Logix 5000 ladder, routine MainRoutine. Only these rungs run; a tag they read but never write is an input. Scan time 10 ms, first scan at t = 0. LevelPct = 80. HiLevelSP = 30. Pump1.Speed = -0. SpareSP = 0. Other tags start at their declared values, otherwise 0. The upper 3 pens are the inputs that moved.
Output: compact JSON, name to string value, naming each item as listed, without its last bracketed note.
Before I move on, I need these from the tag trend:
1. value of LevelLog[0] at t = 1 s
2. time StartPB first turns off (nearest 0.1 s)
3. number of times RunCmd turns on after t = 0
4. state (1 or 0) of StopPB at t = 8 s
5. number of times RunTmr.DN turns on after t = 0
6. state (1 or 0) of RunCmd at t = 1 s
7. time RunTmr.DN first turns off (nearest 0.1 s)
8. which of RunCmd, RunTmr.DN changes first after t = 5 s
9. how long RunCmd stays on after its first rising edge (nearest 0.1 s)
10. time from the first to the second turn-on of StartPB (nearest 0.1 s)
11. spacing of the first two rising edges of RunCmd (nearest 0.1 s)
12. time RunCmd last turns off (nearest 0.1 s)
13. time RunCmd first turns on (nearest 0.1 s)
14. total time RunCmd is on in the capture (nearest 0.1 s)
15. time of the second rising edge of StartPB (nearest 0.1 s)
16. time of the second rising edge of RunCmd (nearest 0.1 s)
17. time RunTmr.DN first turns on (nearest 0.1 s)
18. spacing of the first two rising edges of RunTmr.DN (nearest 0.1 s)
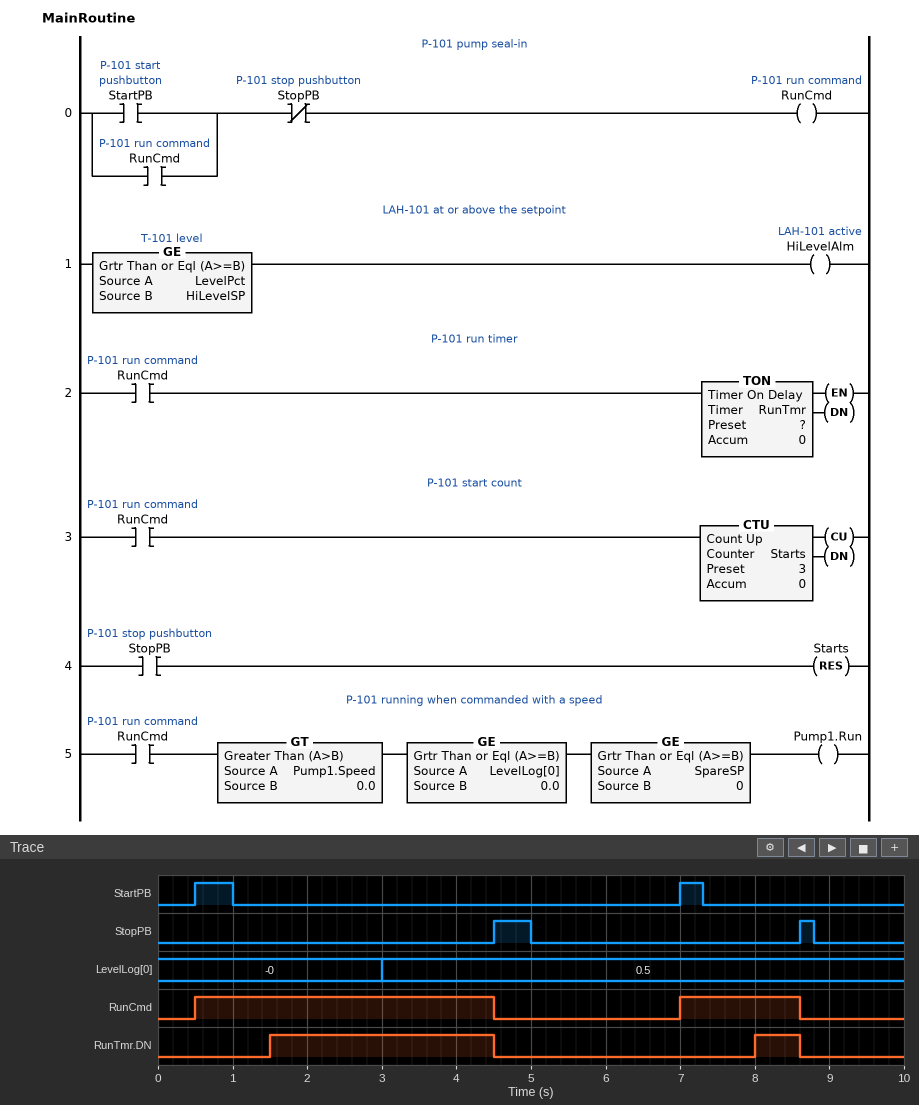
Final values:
{"value of LevelLog[0] at t = 1 s": "-0", "time StartPB first turns off": "1.0 s", "number of times RunCmd turns on after t = 0": "2", "state (1 or 0) of StopPB at t = 8 s": "0", "number of times RunTmr.DN turns on after t = 0": "2", "state (1 or 0) of RunCmd at t = 1 s": "1", "time RunTmr.DN first turns off": "4.5 s", "which of RunCmd, RunTmr.DN changes first after t = 5 s": "RunCmd", "how long RunCmd stays on after its first rising edge": "4.0 s", "time from the first to the second turn-on of StartPB": "6.5 s", "spacing of the first two rising edges of RunCmd": "6.5 s", "time RunCmd last turns off": "8.6 s", "time RunCmd first turns on": "0.5 s", "total time RunCmd is on in the capture": "5.6 s", "time of the second rising edge of StartPB": "7.0 s", "time of the second rising edge of RunCmd": "7.0 s", "time RunTmr.DN first turns on": "1.5 s", "spacing of the first two rising edges of RunTmr.DN": "6.5 s"}
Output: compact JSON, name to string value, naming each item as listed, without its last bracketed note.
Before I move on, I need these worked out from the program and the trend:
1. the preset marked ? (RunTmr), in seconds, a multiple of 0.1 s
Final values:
{"the preset marked ? (RunTmr), in seconds, a multiple of 0.1 s": "1.0 s"}
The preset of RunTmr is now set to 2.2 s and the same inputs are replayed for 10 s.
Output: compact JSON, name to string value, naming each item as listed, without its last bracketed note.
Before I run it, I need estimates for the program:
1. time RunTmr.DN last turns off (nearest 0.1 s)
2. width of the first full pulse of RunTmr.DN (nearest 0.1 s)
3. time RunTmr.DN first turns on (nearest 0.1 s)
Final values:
{"time RunTmr.DN last turns off": "4.5 s", "width of the first full pulse of RunTmr.DN": "1.8 s", "time RunTmr.DN first turns on": "2.7 s"}
